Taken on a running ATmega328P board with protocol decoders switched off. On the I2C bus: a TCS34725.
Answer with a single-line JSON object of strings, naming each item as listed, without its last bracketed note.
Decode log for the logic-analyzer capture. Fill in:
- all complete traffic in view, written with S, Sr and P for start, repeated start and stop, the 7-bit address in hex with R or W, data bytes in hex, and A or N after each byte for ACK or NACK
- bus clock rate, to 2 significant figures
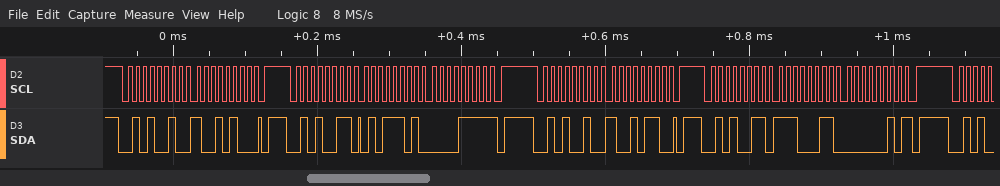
{"all complete traffic in view, written with S, Sr and P for start, repeated start and stop, the 7-bit address in hex with R or W, data bytes in hex, and A or N after each byte for ACK or NACK": "S 29W A 94 A P S 29R A 5D A 0F N P S 29W A 96 A P S 29R A E3 A 02 N P", "bus clock rate, to 2 significant figures": "100 kHz"}
